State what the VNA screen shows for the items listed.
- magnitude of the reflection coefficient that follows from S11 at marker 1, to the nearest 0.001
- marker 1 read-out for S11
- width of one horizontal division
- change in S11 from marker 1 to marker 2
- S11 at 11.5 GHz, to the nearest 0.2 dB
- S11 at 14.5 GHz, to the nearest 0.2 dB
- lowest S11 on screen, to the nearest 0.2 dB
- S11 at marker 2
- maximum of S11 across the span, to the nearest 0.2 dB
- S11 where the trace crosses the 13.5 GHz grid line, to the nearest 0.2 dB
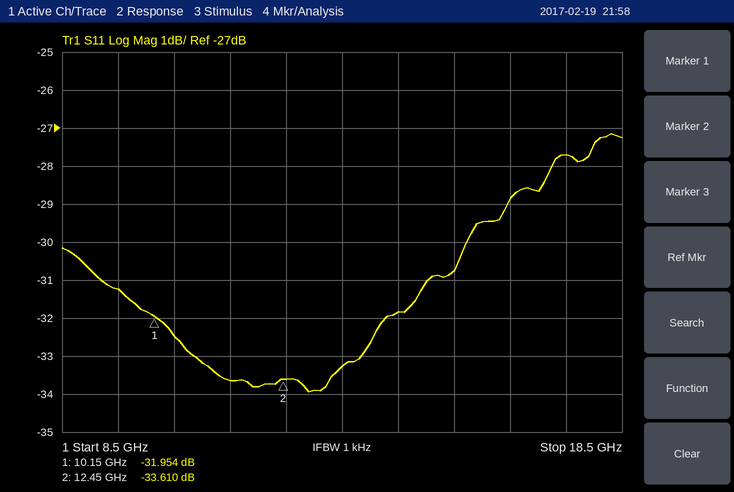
0.025
-31.954 dB
1 GHz
-1.656 dB
-33.6 dB
-31.8 dB
-34.0 dB
-33.610 dB
-27.2 dB
-33.2 dB
